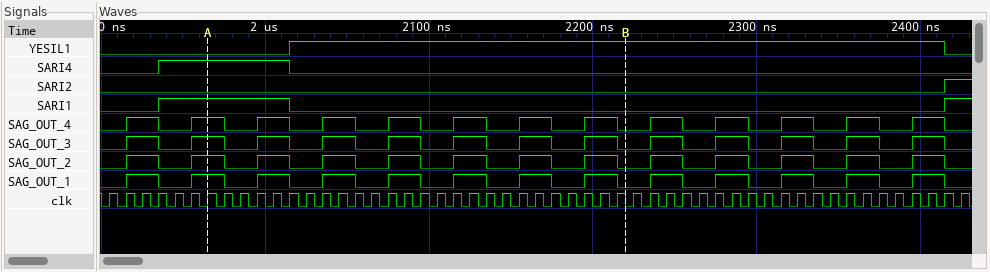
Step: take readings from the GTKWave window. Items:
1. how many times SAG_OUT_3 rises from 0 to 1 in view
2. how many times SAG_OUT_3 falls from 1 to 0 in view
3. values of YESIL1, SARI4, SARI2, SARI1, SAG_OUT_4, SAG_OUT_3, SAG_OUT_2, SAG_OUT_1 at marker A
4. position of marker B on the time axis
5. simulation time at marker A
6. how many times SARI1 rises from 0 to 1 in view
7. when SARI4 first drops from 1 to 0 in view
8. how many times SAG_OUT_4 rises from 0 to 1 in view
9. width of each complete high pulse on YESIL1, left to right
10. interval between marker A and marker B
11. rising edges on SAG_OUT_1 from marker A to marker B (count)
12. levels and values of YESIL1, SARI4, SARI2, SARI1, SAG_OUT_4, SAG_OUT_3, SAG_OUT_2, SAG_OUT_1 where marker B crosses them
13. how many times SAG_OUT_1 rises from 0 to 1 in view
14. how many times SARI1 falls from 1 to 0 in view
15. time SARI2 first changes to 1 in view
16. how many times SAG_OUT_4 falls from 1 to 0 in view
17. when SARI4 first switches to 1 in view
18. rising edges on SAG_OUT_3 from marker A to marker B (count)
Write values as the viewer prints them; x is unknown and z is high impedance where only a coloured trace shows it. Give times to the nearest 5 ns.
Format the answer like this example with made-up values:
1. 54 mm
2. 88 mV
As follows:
1. 13
2. 13
3. YESIL1=0, SARI4=1, SARI2=0, SARI1=1, SAG_OUT_4=1, SAG_OUT_3=1, SAG_OUT_2=1, SAG_OUT_1=1
4. 2220 ns
5. 1965 ns
6. 2
7. 2015 ns
8. 13
9. 400 ns
10. 255 ns
11. 6
12. YESIL1=1, SARI4=0, SARI2=0, SARI1=0, SAG_OUT_4=0, SAG_OUT_3=0, SAG_OUT_2=0, SAG_OUT_1=0
13. 13
14. 1
15. 2415 ns
16. 13
17. 1935 ns
18. 6
